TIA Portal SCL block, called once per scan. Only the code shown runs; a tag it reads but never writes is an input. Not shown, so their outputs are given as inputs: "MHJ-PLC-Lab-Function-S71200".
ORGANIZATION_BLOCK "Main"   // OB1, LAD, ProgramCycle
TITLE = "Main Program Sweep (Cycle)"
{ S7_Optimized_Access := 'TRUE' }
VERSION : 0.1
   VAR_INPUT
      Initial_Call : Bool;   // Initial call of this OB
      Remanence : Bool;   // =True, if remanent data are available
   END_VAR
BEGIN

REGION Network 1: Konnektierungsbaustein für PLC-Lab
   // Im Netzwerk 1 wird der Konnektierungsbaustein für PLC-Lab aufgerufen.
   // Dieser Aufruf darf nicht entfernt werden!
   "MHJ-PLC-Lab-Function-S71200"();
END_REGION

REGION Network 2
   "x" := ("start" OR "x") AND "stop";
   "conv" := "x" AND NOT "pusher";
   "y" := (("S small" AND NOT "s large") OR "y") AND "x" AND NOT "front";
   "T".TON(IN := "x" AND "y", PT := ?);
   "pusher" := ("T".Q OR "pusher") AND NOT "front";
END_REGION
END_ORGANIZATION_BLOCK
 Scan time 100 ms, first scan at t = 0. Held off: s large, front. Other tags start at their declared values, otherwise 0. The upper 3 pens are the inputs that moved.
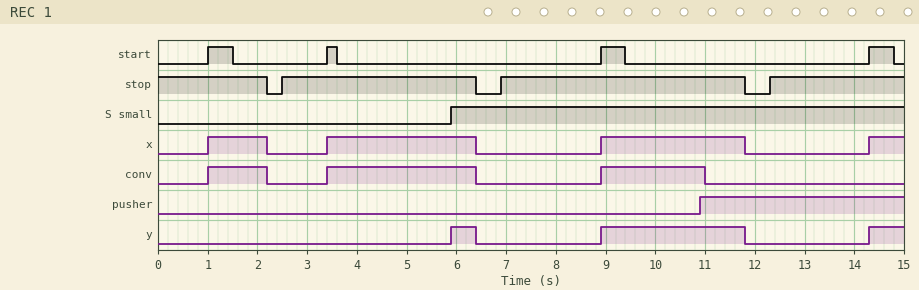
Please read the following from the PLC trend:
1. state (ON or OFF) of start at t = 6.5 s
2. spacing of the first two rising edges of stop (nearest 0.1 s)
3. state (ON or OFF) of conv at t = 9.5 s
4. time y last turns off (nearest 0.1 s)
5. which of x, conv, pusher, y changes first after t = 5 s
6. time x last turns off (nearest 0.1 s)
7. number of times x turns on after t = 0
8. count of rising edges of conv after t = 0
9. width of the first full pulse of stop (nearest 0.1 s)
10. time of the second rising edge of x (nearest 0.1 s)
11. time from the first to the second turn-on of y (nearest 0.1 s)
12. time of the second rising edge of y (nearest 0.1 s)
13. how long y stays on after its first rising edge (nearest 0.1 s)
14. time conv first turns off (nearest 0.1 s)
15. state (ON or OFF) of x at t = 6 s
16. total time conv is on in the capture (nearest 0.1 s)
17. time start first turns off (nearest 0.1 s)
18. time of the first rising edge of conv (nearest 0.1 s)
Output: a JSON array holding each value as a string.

["OFF", "4.4 s", "ON", "11.8 s", "y", "11.8 s", "4", "3", "3.9 s", "3.4 s", "3.0 s", "8.9 s", "0.5 s", "2.2 s", "ON", "6.3 s", "1.5 s", "1.0 s"]
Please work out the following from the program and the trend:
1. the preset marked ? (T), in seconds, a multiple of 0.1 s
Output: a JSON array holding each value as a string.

["2.0 s"]
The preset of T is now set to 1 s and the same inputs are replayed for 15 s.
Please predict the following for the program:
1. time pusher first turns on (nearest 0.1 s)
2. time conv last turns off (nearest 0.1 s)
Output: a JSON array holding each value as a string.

["9.9 s", "10.0 s"]
